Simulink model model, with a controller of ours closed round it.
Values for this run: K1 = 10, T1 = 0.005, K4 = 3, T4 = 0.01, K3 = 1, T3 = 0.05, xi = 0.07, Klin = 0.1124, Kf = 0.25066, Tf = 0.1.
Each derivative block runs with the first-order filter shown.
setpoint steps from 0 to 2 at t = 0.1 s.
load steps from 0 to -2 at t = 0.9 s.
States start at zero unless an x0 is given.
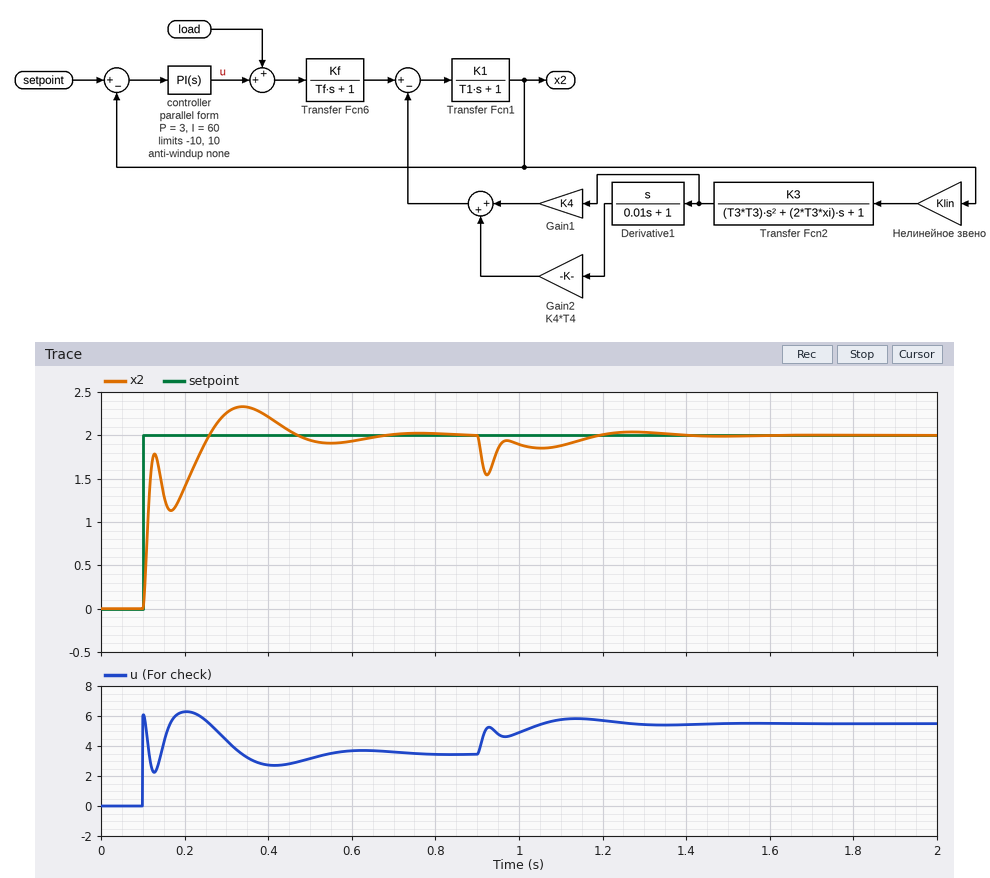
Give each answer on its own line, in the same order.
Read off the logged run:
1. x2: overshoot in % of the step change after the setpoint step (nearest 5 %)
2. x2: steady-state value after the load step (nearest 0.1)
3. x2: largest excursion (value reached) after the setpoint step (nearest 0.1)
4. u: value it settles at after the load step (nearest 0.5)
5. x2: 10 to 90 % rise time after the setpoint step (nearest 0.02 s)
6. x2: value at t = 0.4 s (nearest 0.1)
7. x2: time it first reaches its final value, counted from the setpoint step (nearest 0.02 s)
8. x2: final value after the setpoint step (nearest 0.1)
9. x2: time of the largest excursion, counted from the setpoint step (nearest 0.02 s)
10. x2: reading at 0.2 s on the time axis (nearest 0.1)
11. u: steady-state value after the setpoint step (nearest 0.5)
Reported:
15 %
2.0
2.3
5.5
0.14 s
2.2
0.16 s
2.0
0.24 s
1.4
3.5
